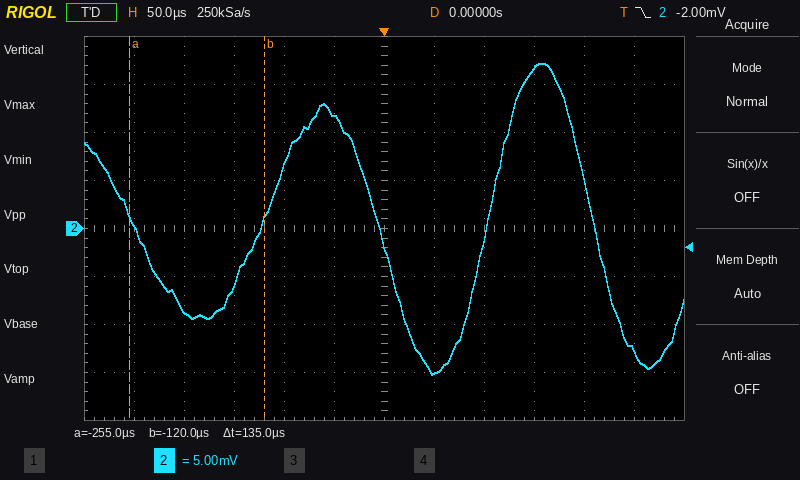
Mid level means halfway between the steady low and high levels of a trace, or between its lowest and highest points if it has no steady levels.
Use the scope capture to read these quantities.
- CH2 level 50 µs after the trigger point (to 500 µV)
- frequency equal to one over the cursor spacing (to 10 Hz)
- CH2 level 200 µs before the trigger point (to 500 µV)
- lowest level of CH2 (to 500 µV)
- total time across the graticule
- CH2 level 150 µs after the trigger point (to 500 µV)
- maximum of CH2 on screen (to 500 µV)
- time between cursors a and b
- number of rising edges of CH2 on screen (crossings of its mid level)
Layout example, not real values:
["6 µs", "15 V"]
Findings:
["-15.0 mV", "7.41 kHz", "-8.5 mV", "-15.0 mV", "600 µs", "16.5 mV", "17.0 mV", "135 µs", "2"]
